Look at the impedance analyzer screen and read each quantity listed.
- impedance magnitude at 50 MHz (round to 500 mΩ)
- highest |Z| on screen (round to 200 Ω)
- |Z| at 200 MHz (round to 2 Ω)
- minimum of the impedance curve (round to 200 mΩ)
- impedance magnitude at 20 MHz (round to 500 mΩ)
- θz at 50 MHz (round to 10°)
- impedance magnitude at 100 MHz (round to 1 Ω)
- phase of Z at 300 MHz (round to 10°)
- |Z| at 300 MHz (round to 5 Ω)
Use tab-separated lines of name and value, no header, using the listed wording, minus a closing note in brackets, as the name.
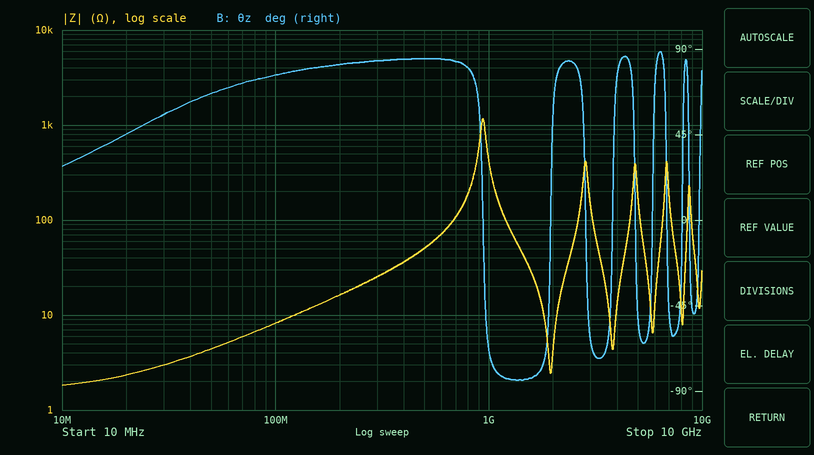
impedance magnitude at 50 MHz	4.5 Ω
highest |Z| on screen	1.2 kΩ
|Z| at 200 MHz	16 Ω
minimum of the impedance curve	1.8 Ω
impedance magnitude at 20 MHz	2.5 Ω
θz at 50 MHz	70°
impedance magnitude at 100 MHz	8 Ω
phase of Z at 300 MHz	80°
|Z| at 300 MHz	25 Ω
